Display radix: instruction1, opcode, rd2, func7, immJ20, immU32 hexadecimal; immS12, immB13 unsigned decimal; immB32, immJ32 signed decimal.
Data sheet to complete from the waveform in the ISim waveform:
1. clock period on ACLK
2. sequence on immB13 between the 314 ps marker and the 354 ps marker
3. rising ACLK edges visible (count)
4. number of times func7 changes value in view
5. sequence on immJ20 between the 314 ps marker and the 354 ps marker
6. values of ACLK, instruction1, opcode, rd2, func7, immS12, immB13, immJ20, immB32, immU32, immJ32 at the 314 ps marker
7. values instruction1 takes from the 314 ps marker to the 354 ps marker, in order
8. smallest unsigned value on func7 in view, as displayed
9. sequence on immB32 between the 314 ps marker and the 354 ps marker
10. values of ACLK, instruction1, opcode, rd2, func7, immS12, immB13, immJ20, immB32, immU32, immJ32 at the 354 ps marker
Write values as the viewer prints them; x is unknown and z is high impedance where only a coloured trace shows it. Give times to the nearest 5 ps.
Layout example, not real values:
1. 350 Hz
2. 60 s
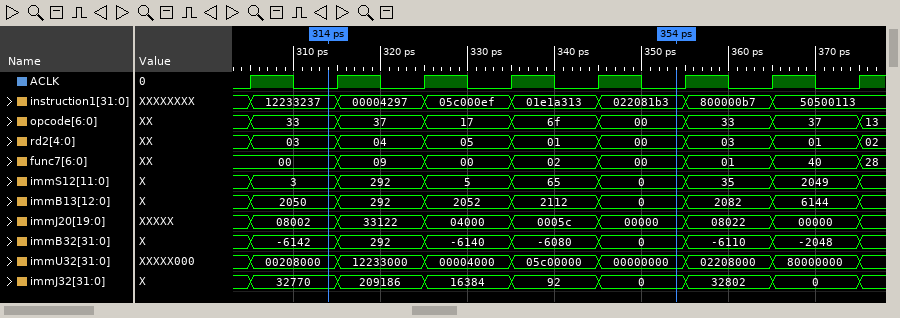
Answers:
1. 10 ps
2. 2050, 292, 2052, 2112, 0
3. 8
4. 7
5. 08002, 33122, 04000, 0005c, 00000
6. ACLK=0, instruction1=12233237, opcode=33, rd2=03, func7=00, immS12=3, immB13=2050, immJ20=08002, immB32=-6142, immU32=00208000, immJ32=32770
7. 12233237, 00004297, 05c000ef, 01e1a313, 022081b3
8. 00
9. -6142, 292, -6140, -6080, 0
10. ACLK=0, instruction1=022081b3, opcode=00, rd2=00, func7=00, immS12=0, immB13=0, immJ20=00000, immB32=0, immU32=00000000, immJ32=0
